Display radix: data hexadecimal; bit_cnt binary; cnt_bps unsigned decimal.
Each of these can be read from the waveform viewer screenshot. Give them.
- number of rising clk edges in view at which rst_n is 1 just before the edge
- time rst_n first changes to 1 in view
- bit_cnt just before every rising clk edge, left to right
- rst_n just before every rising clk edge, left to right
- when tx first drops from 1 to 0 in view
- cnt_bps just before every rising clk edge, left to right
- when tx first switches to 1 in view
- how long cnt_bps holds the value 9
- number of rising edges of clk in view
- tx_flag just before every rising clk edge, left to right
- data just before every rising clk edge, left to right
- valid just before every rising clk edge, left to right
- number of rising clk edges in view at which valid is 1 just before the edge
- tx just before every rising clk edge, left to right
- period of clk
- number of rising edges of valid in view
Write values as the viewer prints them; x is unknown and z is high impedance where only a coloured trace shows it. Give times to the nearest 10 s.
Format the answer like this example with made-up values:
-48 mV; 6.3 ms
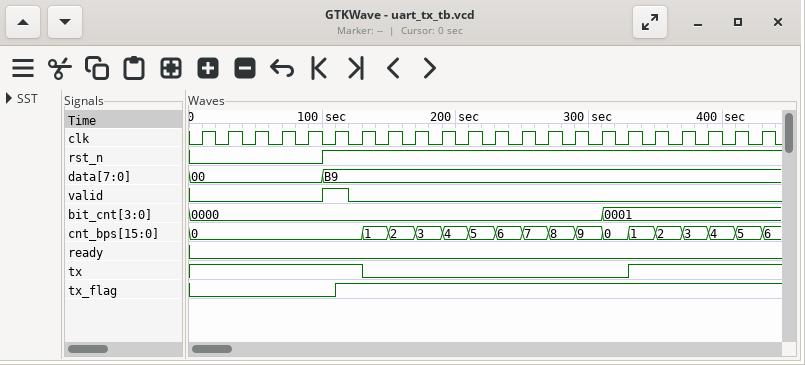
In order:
17; 100 s; 0000, 0000, 0000, 0000, 0000, 0000, 0000, 0000, 0000, 0000, 0000, 0000, 0000, 0000, 0000, 0000, 0001, 0001, 0001, 0001, 0001, 0001; 0 0 0 0 0 1 1 1 1 1 1 1 1 1 1 1 1 1 1 1 1 1; 130 s; 0, 0, 0, 0, 0, 0, 0, 1, 2, 3, 4, 5, 6, 7, 8, 9, 0, 1, 2, 3, 4, 5; 330 s; 20 s; 22; 0 0 0 0 0 0 1 1 1 1 1 1 1 1 1 1 1 1 1 1 1 1; 00, 00, 00, 00, 00, B9, B9, B9, B9, B9, B9, B9, B9, B9, B9, B9, B9, B9, B9, B9, B9, B9; 0 0 0 0 0 1 0 0 0 0 0 0 0 0 0 0 0 0 0 0 0 0; 1; 1 1 1 1 1 1 1 0 0 0 0 0 0 0 0 0 0 1 1 1 1 1; 20 s; 1
